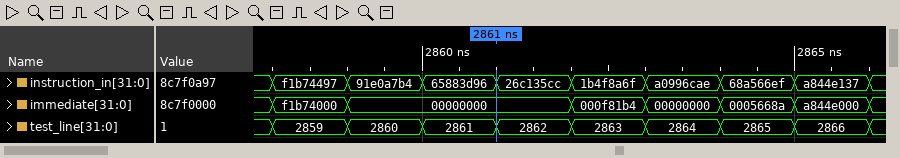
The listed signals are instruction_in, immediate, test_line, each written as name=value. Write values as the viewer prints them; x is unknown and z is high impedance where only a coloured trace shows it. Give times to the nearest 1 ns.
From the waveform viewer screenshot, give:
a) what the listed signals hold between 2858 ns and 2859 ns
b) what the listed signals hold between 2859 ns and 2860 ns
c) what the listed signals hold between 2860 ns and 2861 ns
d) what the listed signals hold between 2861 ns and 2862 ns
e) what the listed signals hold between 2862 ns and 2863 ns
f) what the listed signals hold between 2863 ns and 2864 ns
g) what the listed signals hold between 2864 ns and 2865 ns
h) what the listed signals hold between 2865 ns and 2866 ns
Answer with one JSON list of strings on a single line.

["instruction_in=f1b74497, immediate=f1b74000, test_line=2859", "instruction_in=91e0a7b4, immediate=00000000, test_line=2860", "instruction_in=65883d96, immediate=00000000, test_line=2861", "instruction_in=26c135cc, immediate=00000000, test_line=2862", "instruction_in=1b4f8a6f, immediate=000f81b4, test_line=2863", "instruction_in=a0996cae, immediate=00000000, test_line=2864", "instruction_in=68a566ef, immediate=0005668a, test_line=2865", "instruction_in=a844e137, immediate=a844e000, test_line=2866"]
